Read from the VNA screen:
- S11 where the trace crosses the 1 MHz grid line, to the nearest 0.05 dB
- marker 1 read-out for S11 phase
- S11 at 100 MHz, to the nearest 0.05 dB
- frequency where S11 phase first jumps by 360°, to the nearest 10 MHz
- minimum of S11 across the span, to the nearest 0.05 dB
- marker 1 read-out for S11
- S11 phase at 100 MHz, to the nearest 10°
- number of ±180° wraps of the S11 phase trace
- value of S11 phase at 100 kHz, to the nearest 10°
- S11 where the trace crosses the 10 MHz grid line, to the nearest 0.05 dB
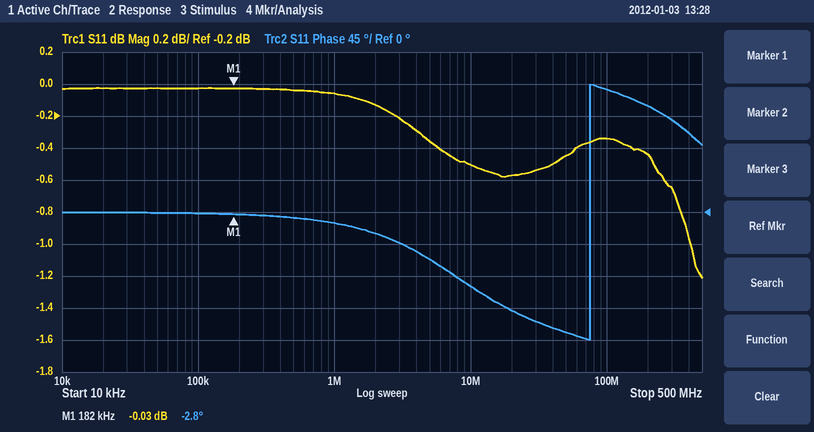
-0.05 dB
-2.8°
-0.35 dB
80 MHz
-1.20 dB
-0.03 dB
170°
1
0°
-0.50 dB
